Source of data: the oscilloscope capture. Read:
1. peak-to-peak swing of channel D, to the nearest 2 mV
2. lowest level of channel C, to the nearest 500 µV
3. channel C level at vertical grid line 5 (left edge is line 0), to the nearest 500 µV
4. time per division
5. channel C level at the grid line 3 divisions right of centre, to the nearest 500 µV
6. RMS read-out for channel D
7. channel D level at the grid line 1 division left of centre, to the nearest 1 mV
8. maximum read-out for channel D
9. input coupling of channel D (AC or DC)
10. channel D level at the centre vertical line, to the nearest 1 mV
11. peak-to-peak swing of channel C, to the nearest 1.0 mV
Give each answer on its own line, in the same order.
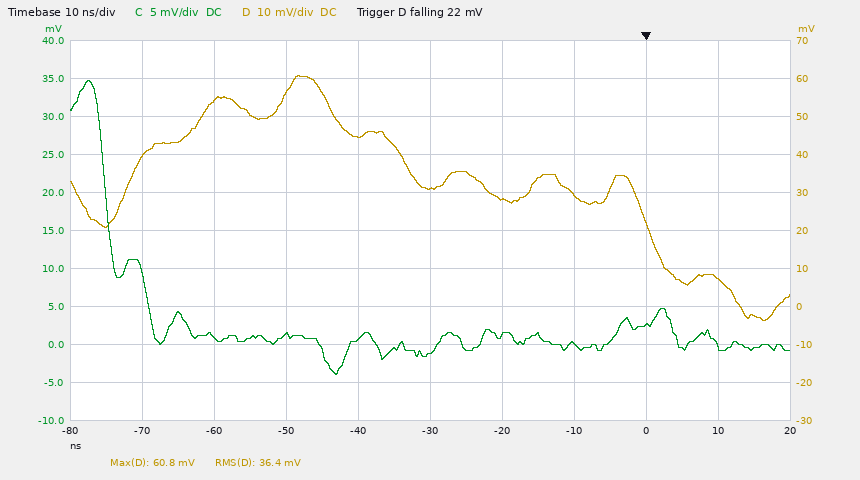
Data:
64 mV
-4.0 mV
-1.0 mV
10 ns
2.5 mV
36.4 mV
45 mV
60.8 mV
DC
31 mV
39.0 mV
